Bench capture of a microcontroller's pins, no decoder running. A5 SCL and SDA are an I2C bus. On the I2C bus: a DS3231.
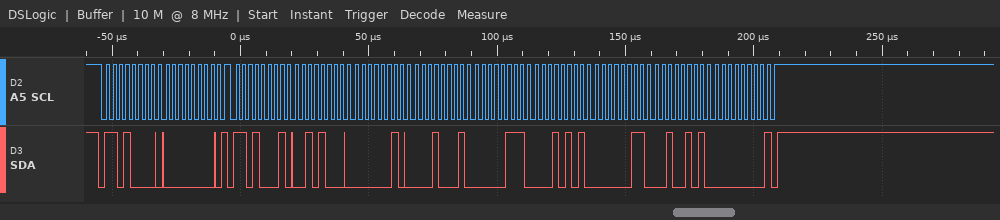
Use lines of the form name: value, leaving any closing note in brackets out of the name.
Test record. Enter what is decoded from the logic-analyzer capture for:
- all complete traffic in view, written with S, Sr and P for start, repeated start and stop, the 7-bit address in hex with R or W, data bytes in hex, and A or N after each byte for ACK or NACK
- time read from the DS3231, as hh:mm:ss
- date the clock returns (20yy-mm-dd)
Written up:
all complete traffic in view, written with S, Sr and P for start, repeated start and stop, the 7-bit address in hex with R or W, data bytes in hex, and A or N after each byte for ACK or NACK: S 68W A 00 A Sr 68R A 28 A 02 A 11 A 07 A 15 A 03 A 25 A 00 N P
time read from the DS3231, as hh:mm:ss: 11:02:28
date the clock returns: 2025-03-15
